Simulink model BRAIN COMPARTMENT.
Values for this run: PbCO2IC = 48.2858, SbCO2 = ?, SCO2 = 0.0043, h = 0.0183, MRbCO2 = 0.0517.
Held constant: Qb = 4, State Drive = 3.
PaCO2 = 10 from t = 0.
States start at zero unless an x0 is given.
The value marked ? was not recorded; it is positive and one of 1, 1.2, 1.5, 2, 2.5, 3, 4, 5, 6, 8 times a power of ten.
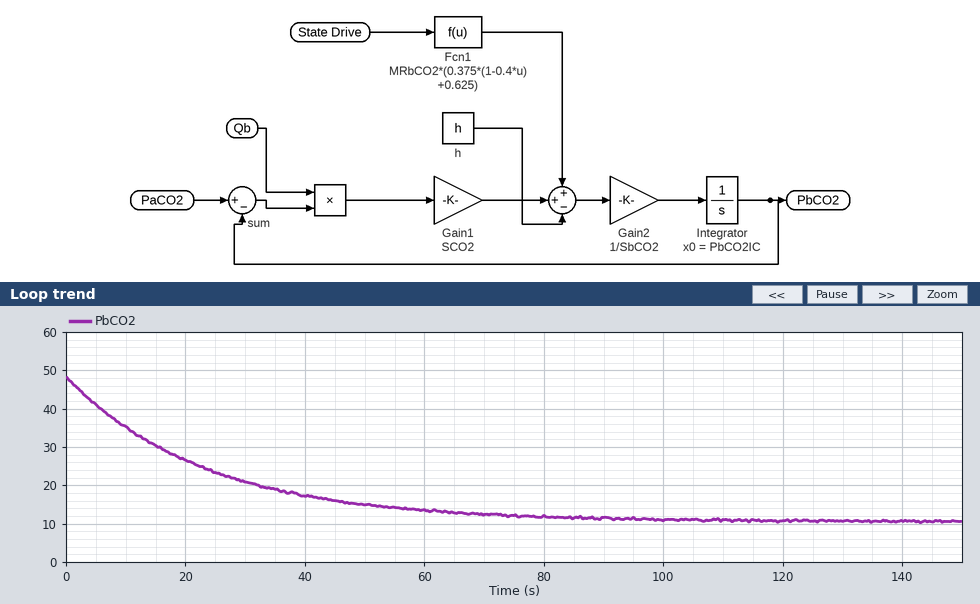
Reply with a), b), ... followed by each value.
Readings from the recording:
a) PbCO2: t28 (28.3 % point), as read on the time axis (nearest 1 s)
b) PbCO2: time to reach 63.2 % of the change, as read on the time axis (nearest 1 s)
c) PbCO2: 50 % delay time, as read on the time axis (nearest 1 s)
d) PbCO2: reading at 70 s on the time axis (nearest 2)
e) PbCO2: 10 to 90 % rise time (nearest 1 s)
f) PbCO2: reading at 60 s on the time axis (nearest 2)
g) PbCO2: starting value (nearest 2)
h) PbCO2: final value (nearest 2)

a) 8 s
b) 23 s
c) 16 s
d) 12
e) 51 s
f) 14
g) 48
h) 10
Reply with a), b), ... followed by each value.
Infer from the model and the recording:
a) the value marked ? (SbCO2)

a) 0.4
